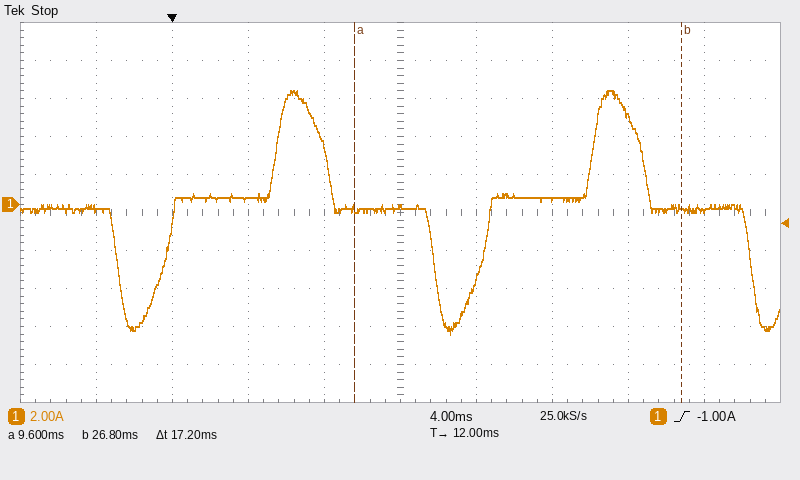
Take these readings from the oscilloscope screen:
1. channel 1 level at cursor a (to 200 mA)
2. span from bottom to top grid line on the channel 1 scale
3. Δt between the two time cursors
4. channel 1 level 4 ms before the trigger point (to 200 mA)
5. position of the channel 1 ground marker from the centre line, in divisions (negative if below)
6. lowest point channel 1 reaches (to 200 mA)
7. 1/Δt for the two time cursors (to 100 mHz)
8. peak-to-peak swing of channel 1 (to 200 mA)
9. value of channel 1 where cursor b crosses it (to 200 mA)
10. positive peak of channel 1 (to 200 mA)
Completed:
-200 mA
20 A
17.2 ms
-200 mA
+0.2 div
-6.8 A
58.1 Hz
12.8 A
-200 mA
6.0 A
